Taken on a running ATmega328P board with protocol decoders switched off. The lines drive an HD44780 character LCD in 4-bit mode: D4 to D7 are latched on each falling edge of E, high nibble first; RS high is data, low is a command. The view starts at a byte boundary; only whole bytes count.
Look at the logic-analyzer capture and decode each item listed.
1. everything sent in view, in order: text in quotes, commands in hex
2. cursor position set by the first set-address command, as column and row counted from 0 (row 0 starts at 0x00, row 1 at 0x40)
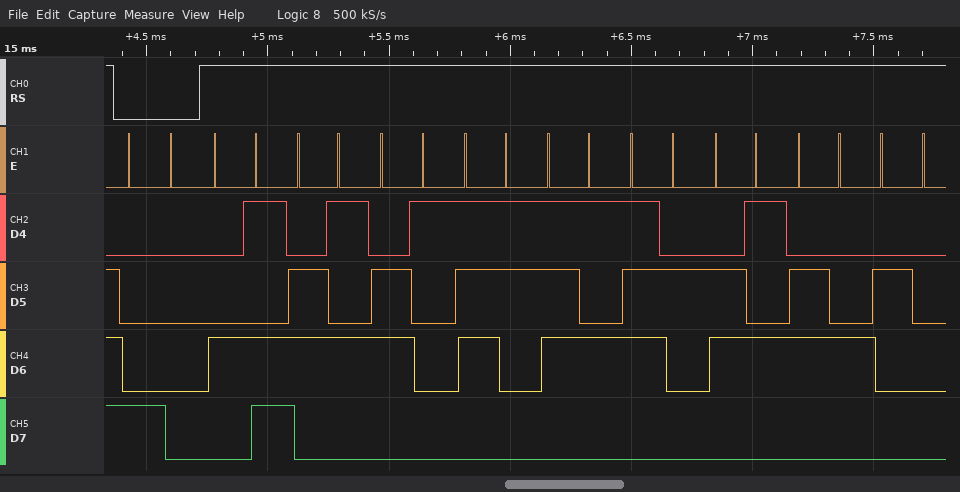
0x80 "Measured "
column 0, row 0
